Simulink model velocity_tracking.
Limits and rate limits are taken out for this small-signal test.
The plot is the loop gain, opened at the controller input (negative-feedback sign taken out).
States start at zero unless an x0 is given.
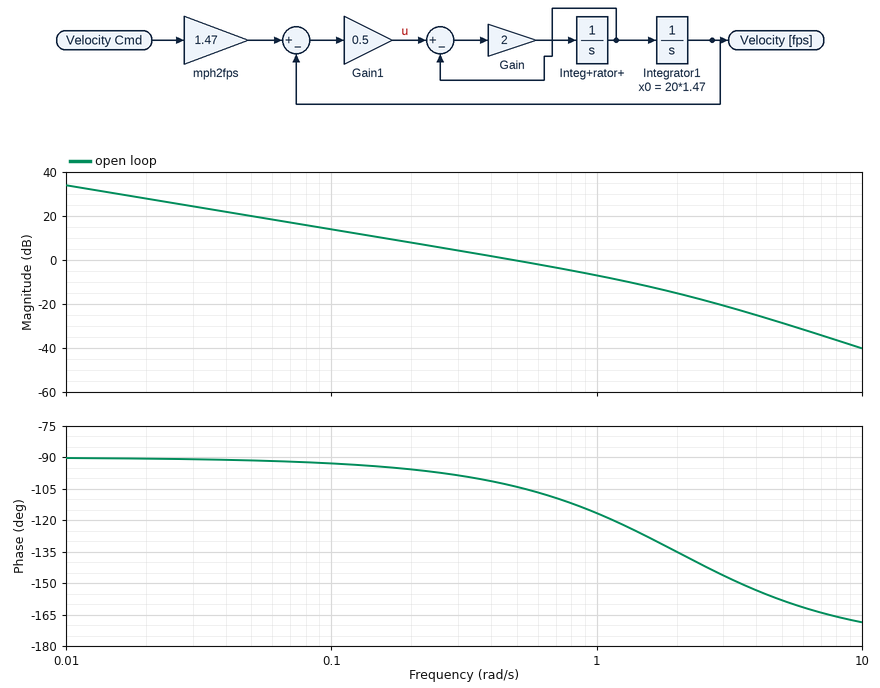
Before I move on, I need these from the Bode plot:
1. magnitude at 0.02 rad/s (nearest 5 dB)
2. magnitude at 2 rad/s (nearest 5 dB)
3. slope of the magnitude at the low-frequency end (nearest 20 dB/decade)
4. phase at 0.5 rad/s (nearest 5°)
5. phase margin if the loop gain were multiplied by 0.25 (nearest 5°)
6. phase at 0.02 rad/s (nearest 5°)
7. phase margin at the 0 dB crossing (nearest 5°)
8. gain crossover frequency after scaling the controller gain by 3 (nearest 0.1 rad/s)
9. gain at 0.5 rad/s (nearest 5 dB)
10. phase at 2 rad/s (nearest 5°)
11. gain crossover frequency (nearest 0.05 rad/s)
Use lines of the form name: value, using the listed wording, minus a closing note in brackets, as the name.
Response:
magnitude at 0.02 rad/s: 30 dB
magnitude at 2 rad/s: -15 dB
slope of the magnitude at the low-frequency end: -20 dB/decade
phase at 0.5 rad/s: -105°
phase margin if the loop gain were multiplied by 0.25: 85°
phase at 0.02 rad/s: -90°
phase margin at the 0 dB crossing: 75°
gain crossover frequency after scaling the controller gain by 3: 1.3 rad/s
gain at 0.5 rad/s: 0 dB
phase at 2 rad/s: -135°
gain crossover frequency: 0.50 rad/s
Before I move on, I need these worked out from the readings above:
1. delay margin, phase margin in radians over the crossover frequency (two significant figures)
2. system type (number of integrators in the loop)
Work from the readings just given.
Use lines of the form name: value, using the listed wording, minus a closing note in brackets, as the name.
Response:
delay margin, phase margin in radians over the crossover frequency: 2.6 s
system type: 1
